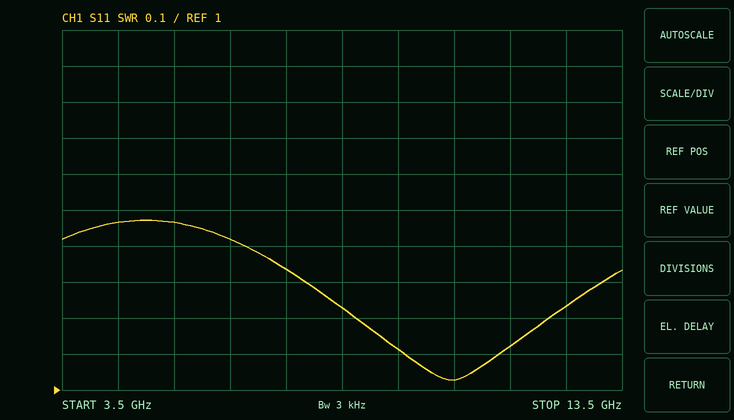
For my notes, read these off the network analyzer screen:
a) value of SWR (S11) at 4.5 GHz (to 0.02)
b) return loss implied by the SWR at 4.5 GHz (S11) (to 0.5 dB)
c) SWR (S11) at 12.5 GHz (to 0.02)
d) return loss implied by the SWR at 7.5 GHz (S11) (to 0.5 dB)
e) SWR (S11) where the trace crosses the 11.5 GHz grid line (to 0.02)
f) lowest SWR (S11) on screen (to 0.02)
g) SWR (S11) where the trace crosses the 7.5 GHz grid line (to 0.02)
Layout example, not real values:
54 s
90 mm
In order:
1.46
14.5 dB
1.24
17.0 dB
1.12
1.02
1.34
